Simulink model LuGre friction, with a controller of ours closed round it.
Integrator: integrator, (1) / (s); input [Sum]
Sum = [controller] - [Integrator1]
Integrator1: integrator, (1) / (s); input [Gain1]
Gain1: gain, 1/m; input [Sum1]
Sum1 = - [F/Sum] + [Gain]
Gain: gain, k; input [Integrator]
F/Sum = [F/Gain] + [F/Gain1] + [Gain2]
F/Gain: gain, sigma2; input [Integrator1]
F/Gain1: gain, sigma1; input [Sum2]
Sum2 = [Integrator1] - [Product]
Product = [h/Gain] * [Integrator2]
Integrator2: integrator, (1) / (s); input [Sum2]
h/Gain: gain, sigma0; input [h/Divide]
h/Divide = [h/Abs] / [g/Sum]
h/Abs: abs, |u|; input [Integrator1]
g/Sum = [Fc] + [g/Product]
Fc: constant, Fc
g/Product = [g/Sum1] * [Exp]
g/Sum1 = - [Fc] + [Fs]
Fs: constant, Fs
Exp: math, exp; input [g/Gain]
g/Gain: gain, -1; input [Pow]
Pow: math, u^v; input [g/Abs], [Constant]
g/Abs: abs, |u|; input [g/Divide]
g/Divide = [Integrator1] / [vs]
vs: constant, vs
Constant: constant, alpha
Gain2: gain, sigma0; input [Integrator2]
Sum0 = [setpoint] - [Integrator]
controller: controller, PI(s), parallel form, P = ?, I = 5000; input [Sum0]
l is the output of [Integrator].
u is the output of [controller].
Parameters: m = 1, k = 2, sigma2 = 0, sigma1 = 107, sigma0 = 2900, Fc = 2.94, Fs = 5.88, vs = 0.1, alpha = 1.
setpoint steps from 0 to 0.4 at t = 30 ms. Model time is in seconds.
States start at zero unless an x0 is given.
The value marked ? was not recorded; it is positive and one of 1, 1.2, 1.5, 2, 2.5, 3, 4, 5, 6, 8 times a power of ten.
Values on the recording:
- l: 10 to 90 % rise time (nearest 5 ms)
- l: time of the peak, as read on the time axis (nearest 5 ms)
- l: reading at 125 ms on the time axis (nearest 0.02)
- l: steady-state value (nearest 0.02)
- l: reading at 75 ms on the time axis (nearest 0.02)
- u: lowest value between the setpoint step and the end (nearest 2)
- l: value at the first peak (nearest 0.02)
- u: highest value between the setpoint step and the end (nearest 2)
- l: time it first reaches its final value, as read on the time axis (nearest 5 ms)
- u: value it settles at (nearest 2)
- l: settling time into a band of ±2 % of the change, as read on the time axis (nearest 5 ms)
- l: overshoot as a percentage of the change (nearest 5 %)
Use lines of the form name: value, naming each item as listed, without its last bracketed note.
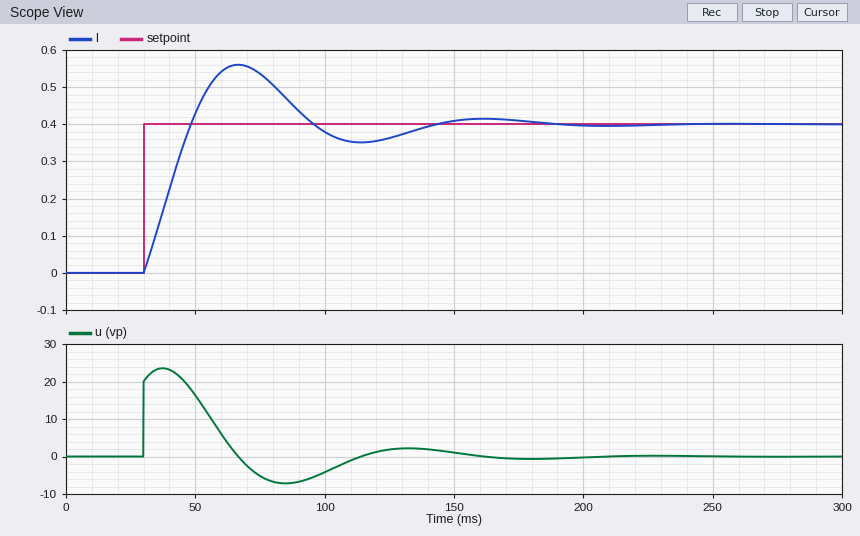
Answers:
l: 10 to 90 % rise time: 15 ms
l: time of the peak, as read on the time axis: 65 ms
l: reading at 125 ms on the time axis: 0.36
l: steady-state value: 0.40
l: reading at 75 ms on the time axis: 0.54
u: lowest value between the setpoint step and the end: -8
l: value at the first peak: 0.56
u: highest value between the setpoint step and the end: 24
l: time it first reaches its final value, as read on the time axis: 50 ms
u: value it settles at: 0
l: settling time into a band of ±2 % of the change, as read on the time axis: 180 ms
l: overshoot as a percentage of the change: 40 %
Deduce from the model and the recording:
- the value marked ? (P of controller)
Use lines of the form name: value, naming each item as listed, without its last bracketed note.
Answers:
the value marked ?: 50
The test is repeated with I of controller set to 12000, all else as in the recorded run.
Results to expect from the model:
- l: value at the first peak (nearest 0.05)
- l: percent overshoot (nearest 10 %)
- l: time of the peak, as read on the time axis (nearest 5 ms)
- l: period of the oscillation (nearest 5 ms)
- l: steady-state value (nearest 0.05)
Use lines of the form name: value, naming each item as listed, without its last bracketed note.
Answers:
l: value at the first peak: 0.60
l: percent overshoot: 50 %
l: time of the peak, as read on the time axis: 55 ms
l: period of the oscillation: 60 ms
l: steady-state value: 0.40
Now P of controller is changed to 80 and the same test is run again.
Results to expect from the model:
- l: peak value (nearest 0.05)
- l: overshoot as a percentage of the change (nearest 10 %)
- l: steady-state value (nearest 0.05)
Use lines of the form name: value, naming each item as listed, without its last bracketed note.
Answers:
l: peak value: 0.50
l: overshoot as a percentage of the change: 30 %
l: steady-state value: 0.40
